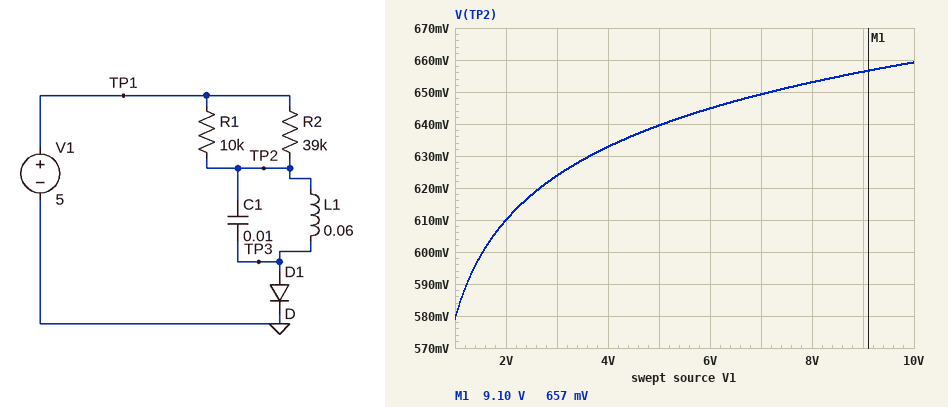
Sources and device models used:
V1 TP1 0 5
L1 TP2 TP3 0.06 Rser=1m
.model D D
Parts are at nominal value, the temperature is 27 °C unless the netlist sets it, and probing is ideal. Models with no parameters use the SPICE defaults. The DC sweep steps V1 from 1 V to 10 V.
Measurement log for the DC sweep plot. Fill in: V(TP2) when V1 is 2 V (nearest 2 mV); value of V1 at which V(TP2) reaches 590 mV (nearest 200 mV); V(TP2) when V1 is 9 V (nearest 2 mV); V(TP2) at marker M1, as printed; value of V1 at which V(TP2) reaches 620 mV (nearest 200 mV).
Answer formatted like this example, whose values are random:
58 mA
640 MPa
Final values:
610 mV
1.2 V
656 mV
657 mV
2.6 V
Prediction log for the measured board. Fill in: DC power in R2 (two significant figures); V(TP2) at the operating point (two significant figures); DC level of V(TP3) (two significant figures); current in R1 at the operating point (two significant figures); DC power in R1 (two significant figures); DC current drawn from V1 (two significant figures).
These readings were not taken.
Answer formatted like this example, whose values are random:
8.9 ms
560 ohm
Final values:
490 µW
640 mV
640 mV
440 µA
1.9 mW
550 µA
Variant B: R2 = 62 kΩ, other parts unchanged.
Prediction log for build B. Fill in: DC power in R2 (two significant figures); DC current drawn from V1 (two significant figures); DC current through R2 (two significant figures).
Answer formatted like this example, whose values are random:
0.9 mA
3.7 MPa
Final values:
310 µW
510 µA
70 µA
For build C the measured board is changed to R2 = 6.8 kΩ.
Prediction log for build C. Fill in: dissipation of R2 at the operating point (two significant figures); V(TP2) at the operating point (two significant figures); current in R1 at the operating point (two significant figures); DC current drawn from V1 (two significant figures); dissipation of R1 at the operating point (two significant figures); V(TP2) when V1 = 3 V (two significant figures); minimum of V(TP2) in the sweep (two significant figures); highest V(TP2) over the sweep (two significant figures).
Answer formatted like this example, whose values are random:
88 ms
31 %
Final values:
2.8 mW
660 mV
430 µA
1.1 mA
1.9 mW
640 mV
600 mV
680 mV
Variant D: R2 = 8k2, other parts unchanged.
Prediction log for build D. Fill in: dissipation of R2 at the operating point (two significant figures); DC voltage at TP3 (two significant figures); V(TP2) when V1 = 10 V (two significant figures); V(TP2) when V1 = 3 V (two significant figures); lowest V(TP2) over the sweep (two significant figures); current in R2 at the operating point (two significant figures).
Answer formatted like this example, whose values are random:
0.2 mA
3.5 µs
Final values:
2.3 mW
650 mV
670 mV
640 mV
590 mV
530 µA
